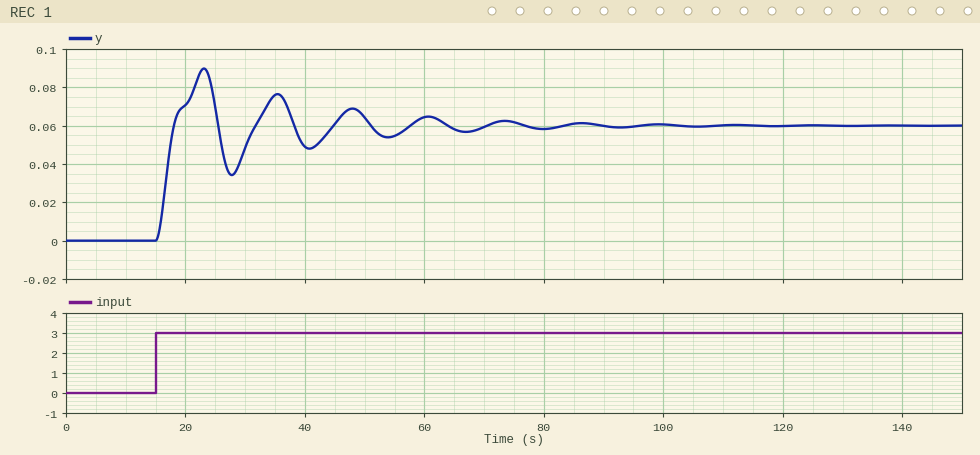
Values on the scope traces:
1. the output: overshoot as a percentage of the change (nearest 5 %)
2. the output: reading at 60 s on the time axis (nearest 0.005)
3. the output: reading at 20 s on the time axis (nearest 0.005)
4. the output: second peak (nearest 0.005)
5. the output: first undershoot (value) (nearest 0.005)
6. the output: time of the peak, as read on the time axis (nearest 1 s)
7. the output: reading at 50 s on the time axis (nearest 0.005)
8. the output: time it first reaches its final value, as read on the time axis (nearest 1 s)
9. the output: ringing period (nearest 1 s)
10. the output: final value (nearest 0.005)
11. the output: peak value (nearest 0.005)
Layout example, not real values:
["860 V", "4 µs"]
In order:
["50 %", "0.065", "0.070", "0.075", "0.035", "23 s", "0.065", "18 s", "12 s", "0.060", "0.090"]
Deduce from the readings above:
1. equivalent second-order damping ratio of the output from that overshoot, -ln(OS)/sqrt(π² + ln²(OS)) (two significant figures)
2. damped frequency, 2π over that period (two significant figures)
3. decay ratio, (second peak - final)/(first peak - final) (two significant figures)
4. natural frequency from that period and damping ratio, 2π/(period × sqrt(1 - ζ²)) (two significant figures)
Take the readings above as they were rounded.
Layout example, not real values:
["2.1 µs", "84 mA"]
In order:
["0.22", "0.52 rad/s", "0.50", "0.54 rad/s"]
